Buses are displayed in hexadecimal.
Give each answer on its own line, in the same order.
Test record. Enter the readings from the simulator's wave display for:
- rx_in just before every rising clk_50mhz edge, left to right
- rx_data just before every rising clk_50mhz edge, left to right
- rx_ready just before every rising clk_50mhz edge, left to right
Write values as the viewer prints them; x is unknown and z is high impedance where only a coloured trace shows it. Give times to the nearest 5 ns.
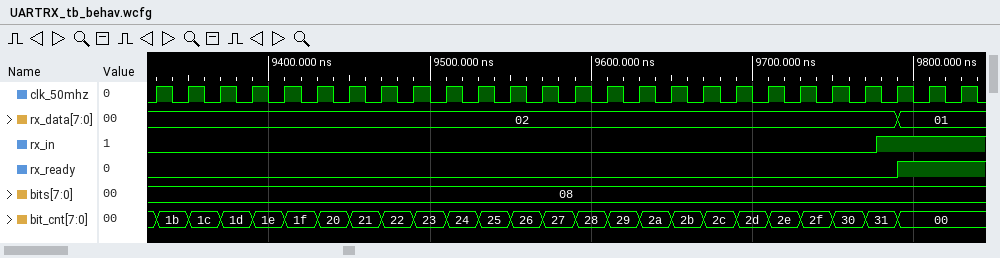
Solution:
0 0 0 0 0 0 0 0 0 0 0 0 0 0 0 0 0 0 0 0 0 0 0 1 1 1
02, 02, 02, 02, 02, 02, 02, 02, 02, 02, 02, 02, 02, 02, 02, 02, 02, 02, 02, 02, 02, 02, 02, 02, 01, 01
0 0 0 0 0 0 0 0 0 0 0 0 0 0 0 0 0 0 0 0 0 0 0 0 1 1
